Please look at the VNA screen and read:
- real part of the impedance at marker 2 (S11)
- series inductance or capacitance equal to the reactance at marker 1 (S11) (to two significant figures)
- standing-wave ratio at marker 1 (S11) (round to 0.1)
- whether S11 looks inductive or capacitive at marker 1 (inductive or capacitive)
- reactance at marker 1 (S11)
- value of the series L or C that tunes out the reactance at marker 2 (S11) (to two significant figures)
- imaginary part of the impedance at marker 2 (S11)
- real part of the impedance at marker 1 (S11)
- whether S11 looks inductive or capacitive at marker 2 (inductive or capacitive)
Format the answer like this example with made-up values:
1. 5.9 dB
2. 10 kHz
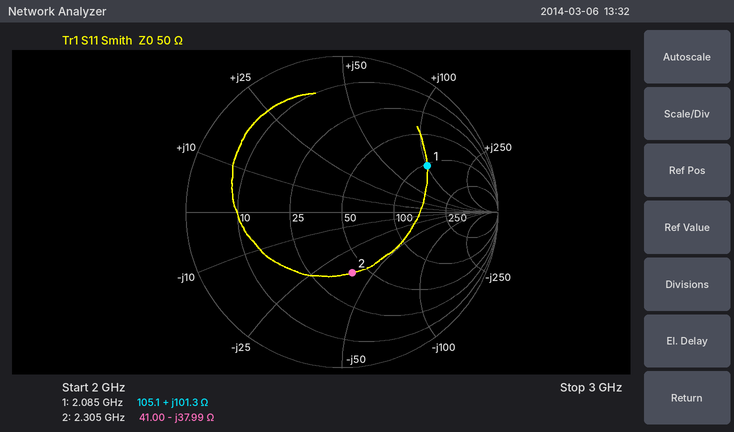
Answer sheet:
1. 41.00 Ω
2. 7.7 nH
3. 4.3
4. inductive
5. +101.3 Ω
6. 2.6 nH
7. -37.99 Ω
8. 105.1 Ω
9. capacitive
